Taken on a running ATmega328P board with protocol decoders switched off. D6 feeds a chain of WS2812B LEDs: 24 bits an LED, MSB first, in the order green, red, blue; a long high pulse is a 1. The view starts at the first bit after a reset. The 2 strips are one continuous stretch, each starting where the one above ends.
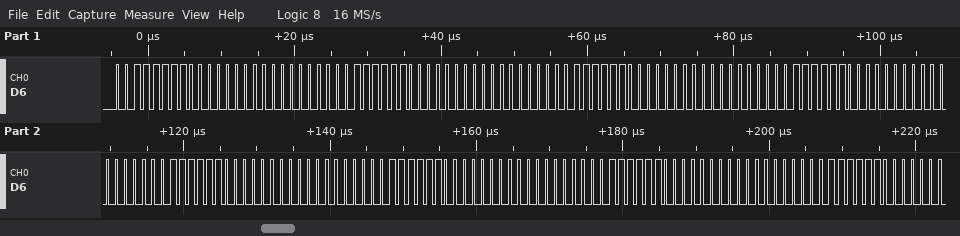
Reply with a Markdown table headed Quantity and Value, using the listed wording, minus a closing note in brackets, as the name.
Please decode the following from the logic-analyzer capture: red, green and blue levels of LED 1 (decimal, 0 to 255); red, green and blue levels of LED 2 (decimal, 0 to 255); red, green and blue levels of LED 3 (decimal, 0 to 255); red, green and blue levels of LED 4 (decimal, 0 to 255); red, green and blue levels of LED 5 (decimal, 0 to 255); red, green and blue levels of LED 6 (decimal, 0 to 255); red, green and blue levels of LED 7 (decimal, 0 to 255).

| Quantity | Value |
|---|---|
| red, green and blue levels of LED 1 | 0, 63, 0 |
| red, green and blue levels of LED 2 | 0, 63, 0 |
| red, green and blue levels of LED 3 | 0, 63, 0 |
| red, green and blue levels of LED 4 | 0, 63, 0 |
| red, green and blue levels of LED 5 | 0, 63, 0 |
| red, green and blue levels of LED 6 | 0, 63, 0 |
| red, green and blue levels of LED 7 | 0, 63, 0 |
